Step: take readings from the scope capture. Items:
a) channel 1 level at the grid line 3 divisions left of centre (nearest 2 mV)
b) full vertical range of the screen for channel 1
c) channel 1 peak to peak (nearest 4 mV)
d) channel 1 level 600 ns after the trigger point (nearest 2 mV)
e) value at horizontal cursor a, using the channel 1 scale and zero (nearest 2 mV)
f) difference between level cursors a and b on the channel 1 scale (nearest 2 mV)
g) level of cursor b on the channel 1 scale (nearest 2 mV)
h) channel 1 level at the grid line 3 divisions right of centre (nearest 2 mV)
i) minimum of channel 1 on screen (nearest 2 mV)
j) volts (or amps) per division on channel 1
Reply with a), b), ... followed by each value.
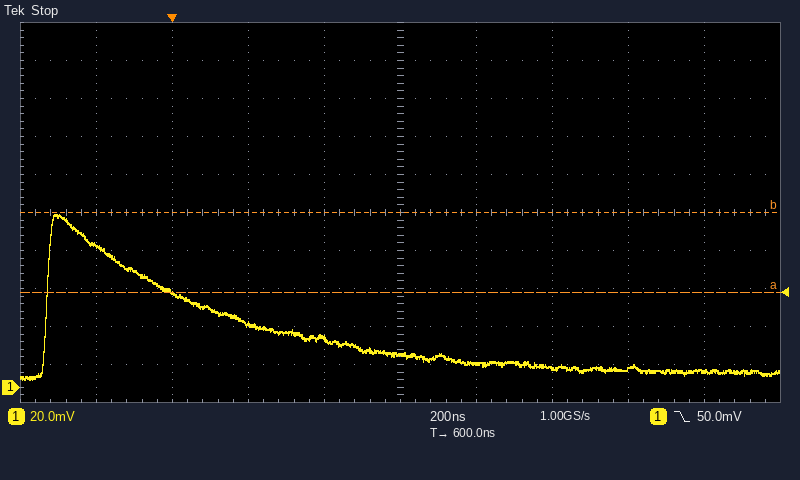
a) 50 mV
b) 200 mV
c) 88 mV
d) 18 mV
e) 50 mV
f) 42 mV
g) 92 mV
h) 10 mV
i) 4 mV
j) 20 mV
